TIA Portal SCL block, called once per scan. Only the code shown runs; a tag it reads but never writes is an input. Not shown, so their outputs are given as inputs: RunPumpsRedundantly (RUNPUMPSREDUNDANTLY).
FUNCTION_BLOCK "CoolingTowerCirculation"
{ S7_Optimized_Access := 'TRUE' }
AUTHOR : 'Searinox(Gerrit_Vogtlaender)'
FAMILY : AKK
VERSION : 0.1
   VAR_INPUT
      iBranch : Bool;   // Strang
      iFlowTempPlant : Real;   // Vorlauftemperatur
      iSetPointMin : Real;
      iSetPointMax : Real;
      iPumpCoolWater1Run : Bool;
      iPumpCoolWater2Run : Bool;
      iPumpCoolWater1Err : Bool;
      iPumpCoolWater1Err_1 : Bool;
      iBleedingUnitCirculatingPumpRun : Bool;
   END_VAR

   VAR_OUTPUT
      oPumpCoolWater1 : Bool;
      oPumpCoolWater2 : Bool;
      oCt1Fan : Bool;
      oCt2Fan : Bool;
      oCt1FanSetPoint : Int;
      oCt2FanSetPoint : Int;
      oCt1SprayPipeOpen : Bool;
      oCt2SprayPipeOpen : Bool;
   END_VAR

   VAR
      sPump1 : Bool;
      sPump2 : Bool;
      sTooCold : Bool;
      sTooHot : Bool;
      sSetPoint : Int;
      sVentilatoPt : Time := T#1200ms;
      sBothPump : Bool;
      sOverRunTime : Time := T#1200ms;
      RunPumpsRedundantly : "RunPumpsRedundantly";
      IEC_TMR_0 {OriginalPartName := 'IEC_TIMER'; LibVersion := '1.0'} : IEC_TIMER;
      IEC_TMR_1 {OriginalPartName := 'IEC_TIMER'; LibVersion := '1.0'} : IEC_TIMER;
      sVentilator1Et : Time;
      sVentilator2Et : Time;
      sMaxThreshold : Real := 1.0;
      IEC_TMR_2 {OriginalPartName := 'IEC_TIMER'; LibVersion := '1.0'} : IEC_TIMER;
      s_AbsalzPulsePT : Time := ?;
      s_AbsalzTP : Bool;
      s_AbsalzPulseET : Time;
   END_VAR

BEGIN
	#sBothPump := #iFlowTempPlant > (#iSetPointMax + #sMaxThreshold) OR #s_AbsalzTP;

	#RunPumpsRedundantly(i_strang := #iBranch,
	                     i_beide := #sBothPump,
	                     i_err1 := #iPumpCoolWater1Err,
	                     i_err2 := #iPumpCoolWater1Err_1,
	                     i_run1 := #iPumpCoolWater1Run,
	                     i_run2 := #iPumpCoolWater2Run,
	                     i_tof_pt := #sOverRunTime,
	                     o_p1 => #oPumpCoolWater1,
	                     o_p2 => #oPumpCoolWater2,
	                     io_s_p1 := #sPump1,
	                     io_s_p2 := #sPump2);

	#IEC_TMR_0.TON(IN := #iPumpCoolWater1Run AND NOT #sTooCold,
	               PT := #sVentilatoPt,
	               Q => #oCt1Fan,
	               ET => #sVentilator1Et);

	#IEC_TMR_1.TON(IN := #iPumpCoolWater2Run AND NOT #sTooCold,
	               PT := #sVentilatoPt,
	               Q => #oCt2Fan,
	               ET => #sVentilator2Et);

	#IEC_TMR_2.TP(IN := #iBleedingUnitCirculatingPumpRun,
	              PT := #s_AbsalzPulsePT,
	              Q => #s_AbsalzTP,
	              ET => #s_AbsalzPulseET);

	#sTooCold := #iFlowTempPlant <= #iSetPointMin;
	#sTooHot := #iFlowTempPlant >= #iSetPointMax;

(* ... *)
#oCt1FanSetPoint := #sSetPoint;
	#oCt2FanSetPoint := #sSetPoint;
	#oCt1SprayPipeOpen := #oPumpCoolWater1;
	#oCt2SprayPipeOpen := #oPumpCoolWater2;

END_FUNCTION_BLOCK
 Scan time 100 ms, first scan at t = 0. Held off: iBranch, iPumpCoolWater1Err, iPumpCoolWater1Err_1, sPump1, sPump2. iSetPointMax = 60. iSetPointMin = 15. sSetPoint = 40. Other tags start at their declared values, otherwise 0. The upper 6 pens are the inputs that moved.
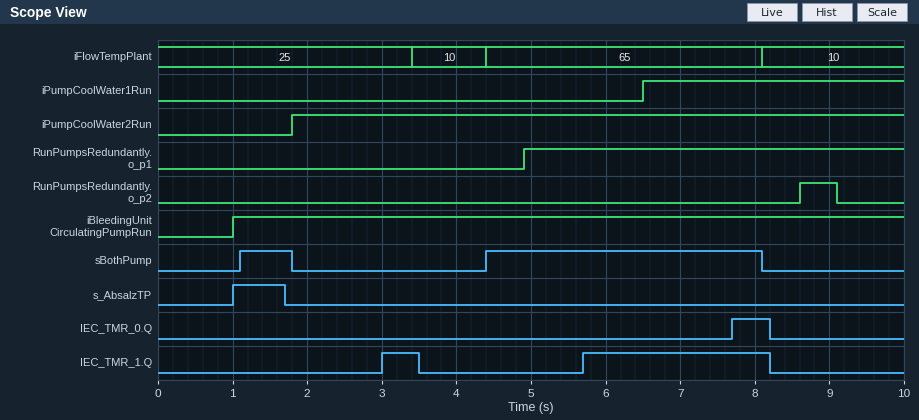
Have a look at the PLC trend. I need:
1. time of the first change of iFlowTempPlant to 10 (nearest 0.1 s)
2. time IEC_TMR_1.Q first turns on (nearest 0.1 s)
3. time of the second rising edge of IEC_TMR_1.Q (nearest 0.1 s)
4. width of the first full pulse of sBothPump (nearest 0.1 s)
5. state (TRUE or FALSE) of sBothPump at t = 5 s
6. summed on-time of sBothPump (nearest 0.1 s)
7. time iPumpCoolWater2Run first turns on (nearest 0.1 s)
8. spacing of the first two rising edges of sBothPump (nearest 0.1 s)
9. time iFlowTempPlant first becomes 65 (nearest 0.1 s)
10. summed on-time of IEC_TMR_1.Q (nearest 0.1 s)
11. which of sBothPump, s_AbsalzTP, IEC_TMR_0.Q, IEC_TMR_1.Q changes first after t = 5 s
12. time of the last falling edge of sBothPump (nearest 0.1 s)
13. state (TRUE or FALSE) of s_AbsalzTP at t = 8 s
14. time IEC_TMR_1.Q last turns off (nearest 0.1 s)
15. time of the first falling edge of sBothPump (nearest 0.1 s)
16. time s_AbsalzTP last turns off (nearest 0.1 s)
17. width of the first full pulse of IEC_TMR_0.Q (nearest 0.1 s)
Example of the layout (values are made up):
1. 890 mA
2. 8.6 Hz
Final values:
1. 3.4 s
2. 3.0 s
3. 5.7 s
4. 0.7 s
5. TRUE
6. 4.4 s
7. 1.8 s
8. 3.3 s
9. 4.4 s
10. 3.0 s
11. IEC_TMR_1.Q
12. 8.1 s
13. FALSE
14. 8.2 s
15. 1.8 s
16. 1.7 s
17. 0.5 s
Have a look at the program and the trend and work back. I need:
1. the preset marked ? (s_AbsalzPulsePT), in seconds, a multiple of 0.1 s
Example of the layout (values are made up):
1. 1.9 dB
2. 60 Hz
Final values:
1. 0.7 s
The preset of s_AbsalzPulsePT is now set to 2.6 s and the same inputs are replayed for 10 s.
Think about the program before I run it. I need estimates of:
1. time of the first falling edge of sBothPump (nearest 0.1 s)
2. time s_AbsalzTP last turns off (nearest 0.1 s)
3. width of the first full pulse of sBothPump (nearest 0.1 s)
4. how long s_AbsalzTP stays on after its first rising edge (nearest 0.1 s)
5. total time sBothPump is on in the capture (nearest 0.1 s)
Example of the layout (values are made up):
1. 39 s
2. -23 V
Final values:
1. 3.7 s
2. 3.6 s
3. 2.6 s
4. 2.6 s
5. 6.3 s
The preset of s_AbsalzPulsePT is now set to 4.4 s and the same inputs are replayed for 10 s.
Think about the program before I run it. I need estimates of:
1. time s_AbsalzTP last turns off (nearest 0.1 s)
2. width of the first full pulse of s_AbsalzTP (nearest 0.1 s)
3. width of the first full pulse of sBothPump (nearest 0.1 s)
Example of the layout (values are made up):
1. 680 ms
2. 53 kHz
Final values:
1. 5.4 s
2. 4.4 s
3. 7.0 s
